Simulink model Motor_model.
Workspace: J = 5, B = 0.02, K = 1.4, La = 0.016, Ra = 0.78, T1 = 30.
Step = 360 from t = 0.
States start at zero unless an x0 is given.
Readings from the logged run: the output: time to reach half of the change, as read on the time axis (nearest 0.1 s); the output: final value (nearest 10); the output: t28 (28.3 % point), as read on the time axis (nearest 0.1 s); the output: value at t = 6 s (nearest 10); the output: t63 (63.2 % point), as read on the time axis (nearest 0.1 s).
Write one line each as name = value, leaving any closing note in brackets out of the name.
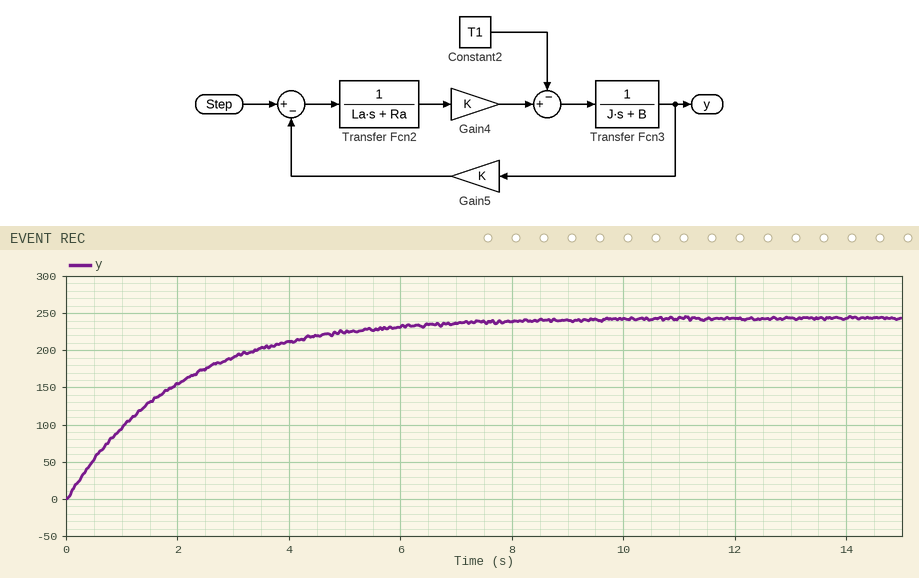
the output: time to reach half of the change, as read on the time axis = 1.4 s
the output: final value = 240
the output: t28 (28.3 % point), as read on the time axis = 0.7 s
the output: value at t = 6 s = 230
the output: t63 (63.2 % point), as read on the time axis = 2.0 s
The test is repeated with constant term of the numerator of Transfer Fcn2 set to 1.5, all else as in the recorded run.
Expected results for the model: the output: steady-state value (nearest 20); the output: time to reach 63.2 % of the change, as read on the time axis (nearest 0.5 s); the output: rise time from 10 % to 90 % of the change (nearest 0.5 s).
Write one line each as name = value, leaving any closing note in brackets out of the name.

the output: steady-state value = 240
the output: time to reach 63.2 % of the change, as read on the time axis = 1.5 s
the output: rise time from 10 % to 90 % of the change = 3.0 s
